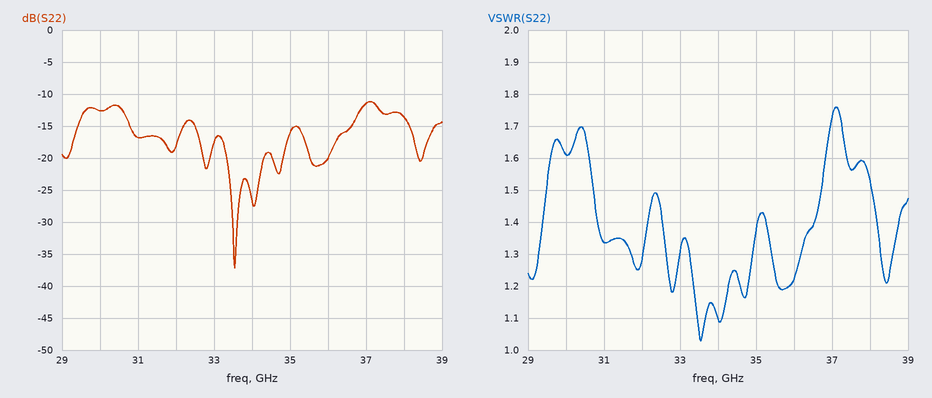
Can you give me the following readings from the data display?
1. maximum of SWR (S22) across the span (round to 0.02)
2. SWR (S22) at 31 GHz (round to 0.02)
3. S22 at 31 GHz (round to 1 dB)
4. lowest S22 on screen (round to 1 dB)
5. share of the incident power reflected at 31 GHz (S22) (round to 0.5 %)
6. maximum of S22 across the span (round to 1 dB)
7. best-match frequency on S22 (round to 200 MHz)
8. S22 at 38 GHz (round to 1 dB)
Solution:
1.76
1.34
-17 dB
-37 dB
2.0 %
-11 dB
33.6 GHz
-14 dB
